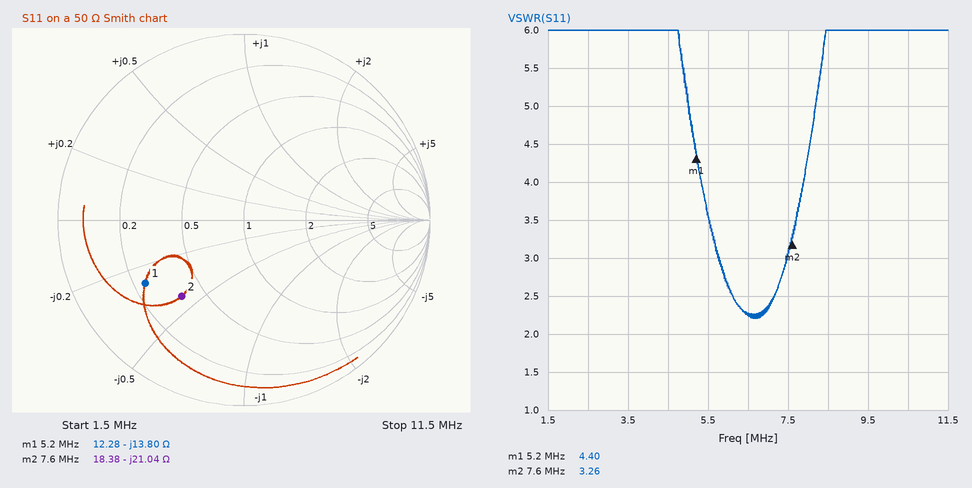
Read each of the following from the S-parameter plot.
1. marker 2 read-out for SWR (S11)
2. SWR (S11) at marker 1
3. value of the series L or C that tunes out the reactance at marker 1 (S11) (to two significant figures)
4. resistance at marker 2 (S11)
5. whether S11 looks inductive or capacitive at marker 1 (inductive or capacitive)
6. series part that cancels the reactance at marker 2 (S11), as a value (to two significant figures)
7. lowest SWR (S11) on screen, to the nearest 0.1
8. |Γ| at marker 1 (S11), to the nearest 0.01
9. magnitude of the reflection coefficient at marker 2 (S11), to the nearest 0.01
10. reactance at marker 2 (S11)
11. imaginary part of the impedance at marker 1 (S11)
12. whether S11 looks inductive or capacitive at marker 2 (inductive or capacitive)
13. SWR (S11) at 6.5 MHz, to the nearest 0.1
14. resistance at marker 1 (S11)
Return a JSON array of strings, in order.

["3.26", "4.40", "420 nH", "18.38 Ω", "capacitive", "440 nH", "2.2", "0.63", "0.53", "-21.04 Ω", "-13.80 Ω", "capacitive", "2.3", "12.28 Ω"]
